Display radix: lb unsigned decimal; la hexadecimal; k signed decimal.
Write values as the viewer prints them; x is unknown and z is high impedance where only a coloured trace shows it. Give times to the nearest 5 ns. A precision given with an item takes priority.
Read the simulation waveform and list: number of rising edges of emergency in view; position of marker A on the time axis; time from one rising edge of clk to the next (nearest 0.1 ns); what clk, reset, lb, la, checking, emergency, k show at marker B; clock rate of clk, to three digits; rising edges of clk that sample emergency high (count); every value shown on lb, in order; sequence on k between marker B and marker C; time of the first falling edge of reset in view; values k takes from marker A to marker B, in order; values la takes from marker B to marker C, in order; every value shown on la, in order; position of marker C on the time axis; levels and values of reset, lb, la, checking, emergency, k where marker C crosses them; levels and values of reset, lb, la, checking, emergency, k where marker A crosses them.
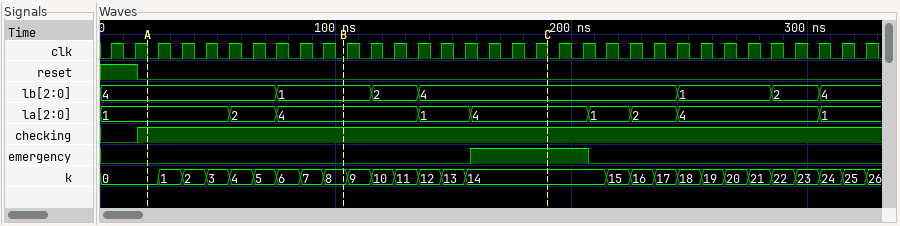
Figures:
1
20 ns
10 ns
clk=0, reset=0, lb=1, la=4, checking=1, emergency=0, k=8
100 MHz
5
4, 1, 2, 4, 1, 2, 4
8, 9, 10, 11, 12, 13, 14
15 ns
0, 1, 2, 3, 4, 5, 6, 7, 8
4, 1, 4
1, 2, 4, 1, 4, 1, 2, 4, 1
190 ns
reset=0, lb=4, la=4, checking=1, emergency=1, k=14
reset=0, lb=4, la=1, checking=1, emergency=0, k=0
